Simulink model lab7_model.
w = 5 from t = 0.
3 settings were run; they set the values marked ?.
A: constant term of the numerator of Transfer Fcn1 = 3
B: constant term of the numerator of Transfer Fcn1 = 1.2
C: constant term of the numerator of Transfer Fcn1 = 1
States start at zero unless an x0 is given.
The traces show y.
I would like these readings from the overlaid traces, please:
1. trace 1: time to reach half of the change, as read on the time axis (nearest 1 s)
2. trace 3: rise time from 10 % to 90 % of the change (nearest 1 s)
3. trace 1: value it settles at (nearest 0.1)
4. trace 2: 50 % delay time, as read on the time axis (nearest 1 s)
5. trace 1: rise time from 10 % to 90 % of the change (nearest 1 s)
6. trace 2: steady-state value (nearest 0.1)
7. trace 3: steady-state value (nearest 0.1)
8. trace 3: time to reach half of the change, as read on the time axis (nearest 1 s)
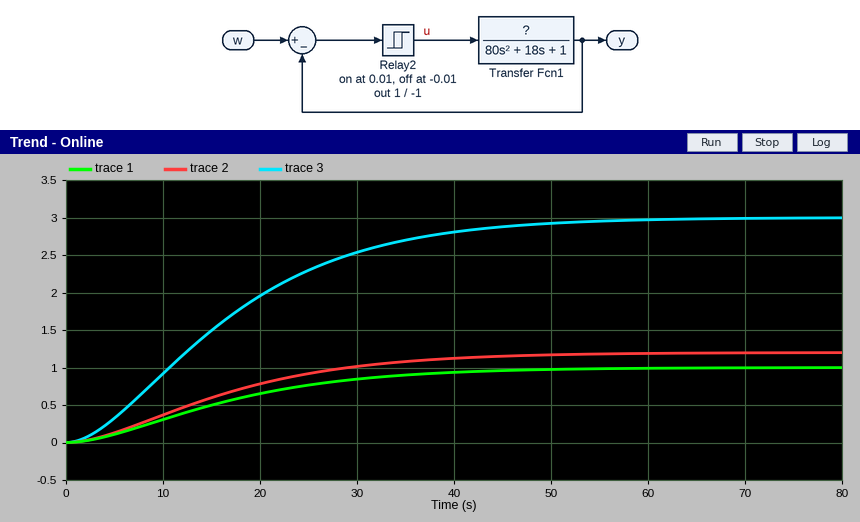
15 s
30 s
1.0
15 s
30 s
1.2
3.0
15 s
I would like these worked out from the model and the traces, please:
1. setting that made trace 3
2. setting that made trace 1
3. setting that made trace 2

A
C
B
